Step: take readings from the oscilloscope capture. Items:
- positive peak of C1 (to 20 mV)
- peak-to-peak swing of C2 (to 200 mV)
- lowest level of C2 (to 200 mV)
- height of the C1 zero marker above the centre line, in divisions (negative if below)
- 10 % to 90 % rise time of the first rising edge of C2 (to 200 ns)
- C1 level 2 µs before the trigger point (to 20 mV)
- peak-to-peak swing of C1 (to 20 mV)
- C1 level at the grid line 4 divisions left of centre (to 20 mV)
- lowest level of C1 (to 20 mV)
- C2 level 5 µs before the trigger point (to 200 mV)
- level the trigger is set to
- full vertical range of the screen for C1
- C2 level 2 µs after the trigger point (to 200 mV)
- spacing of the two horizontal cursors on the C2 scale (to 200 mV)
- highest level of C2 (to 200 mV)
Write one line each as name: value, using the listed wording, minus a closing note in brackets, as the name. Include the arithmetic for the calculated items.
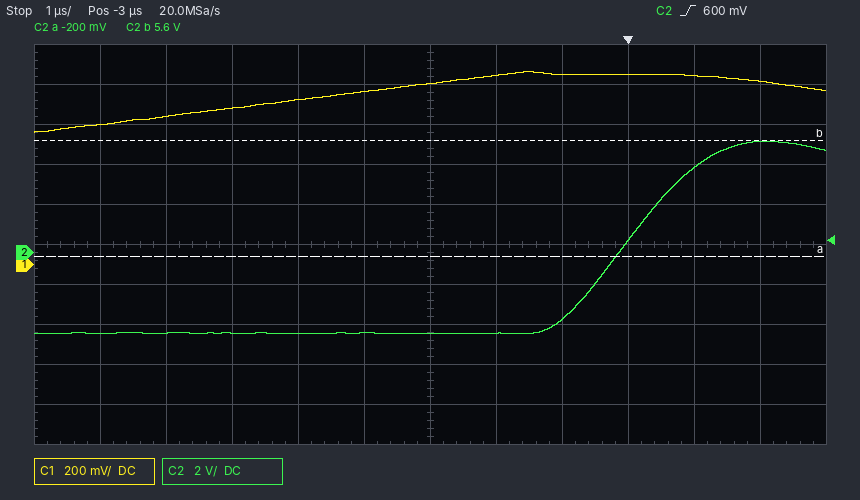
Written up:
positive peak of C1: 960 mV
peak-to-peak swing of C2: 5.6 V − (-4.0 V) = 9.6 V
lowest level of C2: -4.0 V
height of the C1 zero marker above the centre line, in divisions: -0.5 div
10 % to 90 % rise time of the first rising edge of C2: 2.0 µs
C1 level 2 µs before the trigger point: 940 mV
peak-to-peak swing of C1: 960 mV − (660 mV) = 300 mV
C1 level at the grid line 4 divisions left of centre: 740 mV
lowest level of C1: 660 mV
C2 level 5 µs before the trigger point: -4.0 V
level the trigger is set to: 600 mV
full vertical range of the screen for C1: 2 V
C2 level 2 µs after the trigger point: 5.6 V
spacing of the two horizontal cursors on the C2 scale: 5.8 V
highest level of C2: 5.6 V
